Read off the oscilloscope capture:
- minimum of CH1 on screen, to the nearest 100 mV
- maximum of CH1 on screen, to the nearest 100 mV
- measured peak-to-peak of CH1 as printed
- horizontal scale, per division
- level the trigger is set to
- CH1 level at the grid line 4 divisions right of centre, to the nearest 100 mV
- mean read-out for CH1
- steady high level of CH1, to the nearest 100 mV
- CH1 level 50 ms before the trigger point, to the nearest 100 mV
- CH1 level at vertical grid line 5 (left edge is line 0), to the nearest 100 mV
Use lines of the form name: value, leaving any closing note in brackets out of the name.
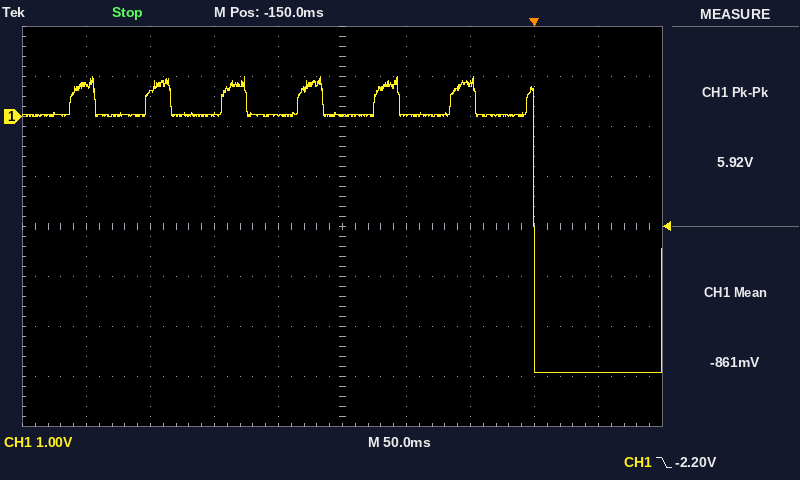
minimum of CH1 on screen, to the nearest 100 mV: -5.1 V
maximum of CH1 on screen, to the nearest 100 mV: 800 mV
measured peak-to-peak of CH1 as printed: 5.92 V
horizontal scale, per division: 50 ms
level the trigger is set to: -2.20 V
CH1 level at the grid line 4 divisions right of centre, to the nearest 100 mV: -5.1 V
mean read-out for CH1: -861 mV
steady high level of CH1, to the nearest 100 mV: 0.0 V
CH1 level 50 ms before the trigger point, to the nearest 100 mV: 700 mV
CH1 level at vertical grid line 5 (left edge is line 0), to the nearest 100 mV: 0.0 V
